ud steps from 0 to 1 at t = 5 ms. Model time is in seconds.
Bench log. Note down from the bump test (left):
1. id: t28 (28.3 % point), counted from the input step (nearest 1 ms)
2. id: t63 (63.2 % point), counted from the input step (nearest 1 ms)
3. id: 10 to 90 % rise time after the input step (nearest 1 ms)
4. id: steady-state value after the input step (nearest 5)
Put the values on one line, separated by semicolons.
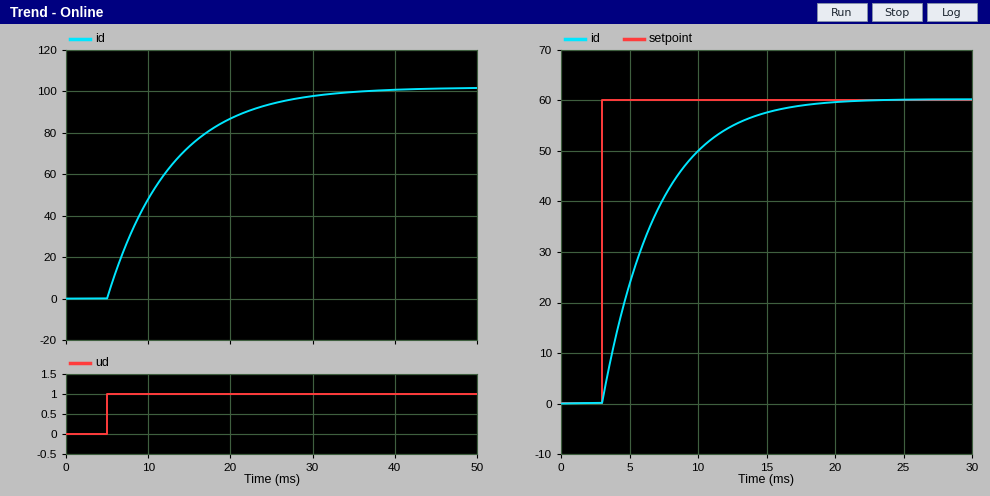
3 ms; 8 ms; 17 ms; 100
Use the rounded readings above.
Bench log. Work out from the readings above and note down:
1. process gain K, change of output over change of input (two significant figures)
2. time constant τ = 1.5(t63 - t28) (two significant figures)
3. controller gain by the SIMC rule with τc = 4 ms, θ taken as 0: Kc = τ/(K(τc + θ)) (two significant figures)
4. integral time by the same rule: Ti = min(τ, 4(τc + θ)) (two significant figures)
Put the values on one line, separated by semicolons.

100; 7.5 ms; 0.019; 7.5 ms
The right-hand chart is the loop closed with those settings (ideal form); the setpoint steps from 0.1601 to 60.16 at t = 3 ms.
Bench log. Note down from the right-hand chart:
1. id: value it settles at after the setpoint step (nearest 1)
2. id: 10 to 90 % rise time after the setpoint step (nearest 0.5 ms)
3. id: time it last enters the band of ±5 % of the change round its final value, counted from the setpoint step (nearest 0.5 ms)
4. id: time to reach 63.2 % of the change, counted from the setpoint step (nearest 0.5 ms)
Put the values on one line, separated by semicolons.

60; 8.5 ms; 11.5 ms; 4.0 ms
